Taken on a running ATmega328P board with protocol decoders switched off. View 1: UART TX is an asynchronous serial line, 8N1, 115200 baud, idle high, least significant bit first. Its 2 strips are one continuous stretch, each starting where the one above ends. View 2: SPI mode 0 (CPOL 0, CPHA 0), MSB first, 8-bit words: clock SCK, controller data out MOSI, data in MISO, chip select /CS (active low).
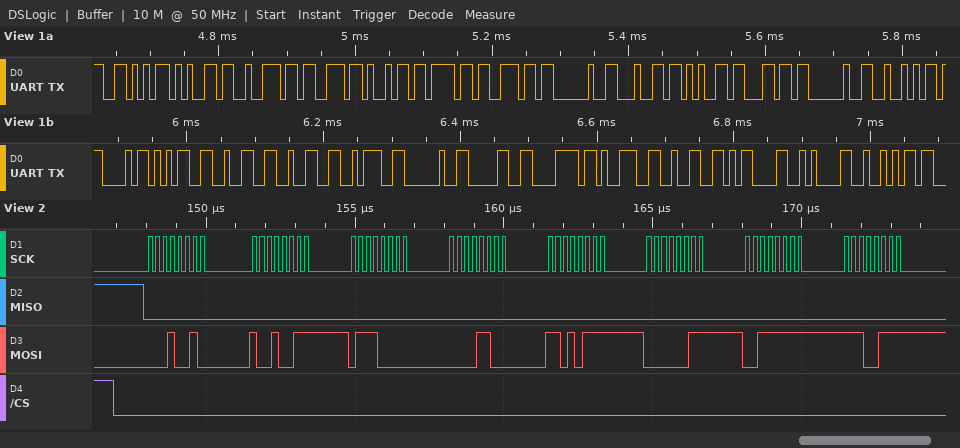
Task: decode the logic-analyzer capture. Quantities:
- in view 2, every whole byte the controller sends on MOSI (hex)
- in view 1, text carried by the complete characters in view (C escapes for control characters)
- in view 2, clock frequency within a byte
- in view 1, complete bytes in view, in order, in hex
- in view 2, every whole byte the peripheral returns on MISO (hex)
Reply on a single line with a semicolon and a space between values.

12 93 70 0C D7 03 3F E7; "Version del RC522: 0x92\r\nR"; 4 MHz; 0x56 0x65 0x72 0x73 0x69 0x6F 0x6E 0x20 0x64 0x65 0x6C 0x20 0x52 0x43 0x35 0x32 0x32 0x3A 0x20 0x30 0x78 0x39 0x32 0x0D 0x0A 0x52; 00 00 00 00 00 00 00 00
